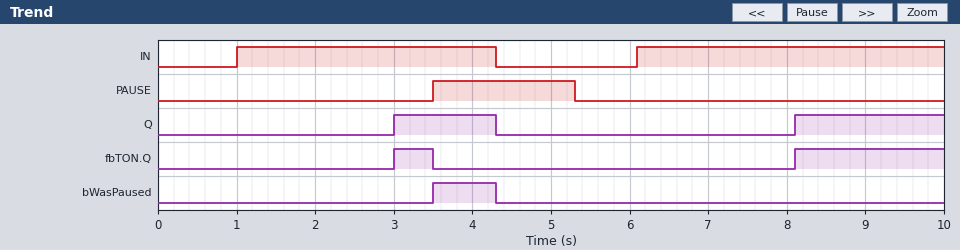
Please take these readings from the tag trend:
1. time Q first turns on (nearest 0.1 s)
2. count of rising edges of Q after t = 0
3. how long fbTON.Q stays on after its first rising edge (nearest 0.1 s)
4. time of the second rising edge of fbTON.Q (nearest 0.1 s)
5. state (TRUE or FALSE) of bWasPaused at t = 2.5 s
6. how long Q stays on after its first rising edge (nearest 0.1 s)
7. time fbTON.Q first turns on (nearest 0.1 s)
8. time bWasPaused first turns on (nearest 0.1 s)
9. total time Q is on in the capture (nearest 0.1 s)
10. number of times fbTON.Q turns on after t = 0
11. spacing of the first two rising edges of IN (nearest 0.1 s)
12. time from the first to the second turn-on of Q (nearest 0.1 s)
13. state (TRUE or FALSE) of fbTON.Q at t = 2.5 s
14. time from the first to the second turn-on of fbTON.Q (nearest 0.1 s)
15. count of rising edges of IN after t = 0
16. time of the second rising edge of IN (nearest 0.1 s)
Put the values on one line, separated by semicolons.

3.0 s; 2; 0.5 s; 8.1 s; FALSE; 1.3 s; 3.0 s; 3.5 s; 3.2 s; 2; 5.1 s; 5.1 s; FALSE; 5.1 s; 2; 6.1 s
